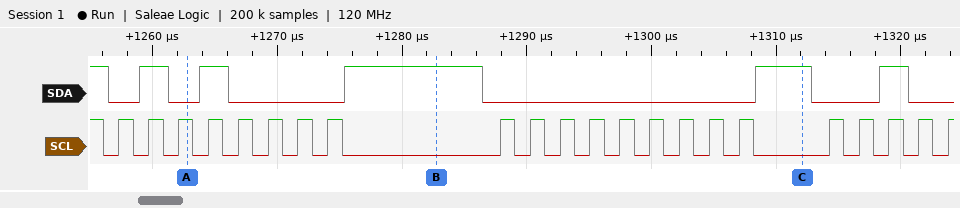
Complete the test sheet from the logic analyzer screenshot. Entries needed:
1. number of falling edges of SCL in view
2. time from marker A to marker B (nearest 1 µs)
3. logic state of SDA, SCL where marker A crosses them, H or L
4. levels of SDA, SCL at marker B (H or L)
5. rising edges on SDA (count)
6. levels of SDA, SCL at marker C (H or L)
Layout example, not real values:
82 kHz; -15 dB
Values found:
22; 20 µs; SDA=L, SCL=H; SDA=H, SCL=L; 5; SDA=H, SCL=L
